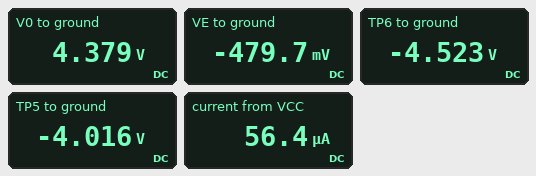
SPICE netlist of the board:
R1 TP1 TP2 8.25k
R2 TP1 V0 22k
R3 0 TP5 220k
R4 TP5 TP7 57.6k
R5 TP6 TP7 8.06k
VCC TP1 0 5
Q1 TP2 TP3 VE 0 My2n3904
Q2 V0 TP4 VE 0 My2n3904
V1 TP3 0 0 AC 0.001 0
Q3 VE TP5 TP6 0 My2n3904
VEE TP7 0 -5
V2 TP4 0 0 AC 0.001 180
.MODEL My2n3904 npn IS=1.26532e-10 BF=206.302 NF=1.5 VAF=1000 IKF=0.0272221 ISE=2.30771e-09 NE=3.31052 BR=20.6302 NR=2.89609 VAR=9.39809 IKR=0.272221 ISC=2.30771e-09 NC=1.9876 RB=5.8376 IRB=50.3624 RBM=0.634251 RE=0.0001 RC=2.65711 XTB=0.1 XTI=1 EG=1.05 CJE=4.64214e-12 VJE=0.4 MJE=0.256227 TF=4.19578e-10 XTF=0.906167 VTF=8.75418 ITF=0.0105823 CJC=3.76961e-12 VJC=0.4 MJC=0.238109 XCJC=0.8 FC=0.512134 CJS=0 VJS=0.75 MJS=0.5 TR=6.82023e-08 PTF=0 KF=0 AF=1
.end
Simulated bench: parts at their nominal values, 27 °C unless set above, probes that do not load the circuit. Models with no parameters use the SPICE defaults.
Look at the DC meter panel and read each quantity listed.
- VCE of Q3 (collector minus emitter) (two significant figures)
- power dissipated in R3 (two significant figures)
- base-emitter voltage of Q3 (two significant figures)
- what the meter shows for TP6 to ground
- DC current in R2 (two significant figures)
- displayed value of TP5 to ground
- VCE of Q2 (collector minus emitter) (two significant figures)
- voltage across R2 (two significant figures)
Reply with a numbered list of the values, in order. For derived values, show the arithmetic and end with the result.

1. -479.7 mV - (-4.523 V) = 4.0 V
2. (0 V - (-4.016 V))^2 / 220 kΩ = 73 µW
3. -4.016 V - (-4.523 V) = 510 mV
4. -4.523 V
5. (5 V - 4.379 V) / 22 kΩ = 28 µA
6. -4.016 V
7. 4.379 V - (-479.7 mV) = 4.9 V
8. 5 V - 4.379 V = 620 mV
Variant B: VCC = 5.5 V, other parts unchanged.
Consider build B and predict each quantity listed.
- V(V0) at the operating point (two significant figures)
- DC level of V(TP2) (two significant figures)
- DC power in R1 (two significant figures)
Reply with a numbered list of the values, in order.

1. 4.9 V
2. 5.3 V
3. 6.6 µW
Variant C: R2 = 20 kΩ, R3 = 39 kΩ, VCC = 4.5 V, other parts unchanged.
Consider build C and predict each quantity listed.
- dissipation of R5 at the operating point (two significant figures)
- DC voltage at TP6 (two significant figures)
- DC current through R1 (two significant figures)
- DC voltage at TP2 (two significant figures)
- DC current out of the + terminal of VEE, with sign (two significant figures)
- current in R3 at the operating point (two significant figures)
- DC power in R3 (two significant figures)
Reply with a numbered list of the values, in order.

1. 680 µW
2. -2.7 V
3. 140 µA
4. 3.3 V
5. -340 µA
6. 54 µA
7. 110 µW
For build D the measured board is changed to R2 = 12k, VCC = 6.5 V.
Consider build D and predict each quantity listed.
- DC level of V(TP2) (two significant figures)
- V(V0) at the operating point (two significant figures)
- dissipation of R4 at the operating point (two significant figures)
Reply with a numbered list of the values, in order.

1. 6.3 V
2. 6.2 V
3. 17 µW
